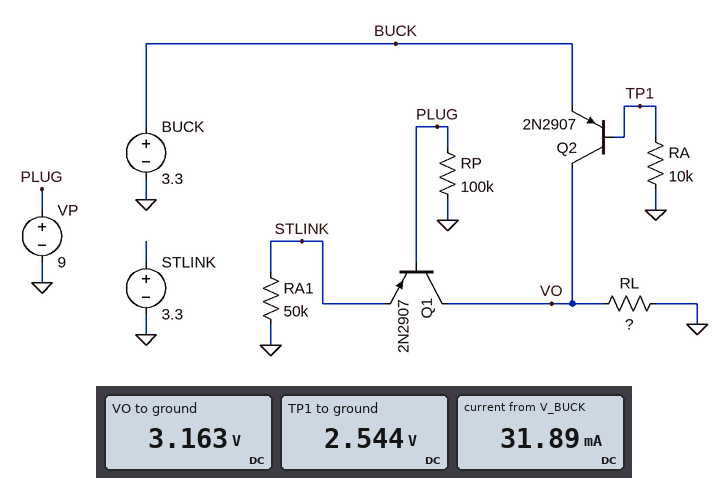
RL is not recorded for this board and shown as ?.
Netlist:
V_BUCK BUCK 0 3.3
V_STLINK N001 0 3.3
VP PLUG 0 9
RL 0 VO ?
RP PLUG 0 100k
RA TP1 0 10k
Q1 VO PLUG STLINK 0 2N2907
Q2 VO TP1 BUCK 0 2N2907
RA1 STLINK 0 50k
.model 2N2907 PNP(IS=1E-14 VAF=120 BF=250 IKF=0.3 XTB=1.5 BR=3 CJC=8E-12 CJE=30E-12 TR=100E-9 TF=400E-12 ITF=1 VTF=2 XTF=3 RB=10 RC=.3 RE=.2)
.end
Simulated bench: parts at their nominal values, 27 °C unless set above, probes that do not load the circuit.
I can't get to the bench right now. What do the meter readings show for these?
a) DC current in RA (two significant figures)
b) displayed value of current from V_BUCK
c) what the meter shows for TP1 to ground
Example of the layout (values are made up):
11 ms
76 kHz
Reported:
250 µA
31.89 mA
2.544 V
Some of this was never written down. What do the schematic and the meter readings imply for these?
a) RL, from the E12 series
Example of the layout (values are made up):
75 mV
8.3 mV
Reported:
100 Ω
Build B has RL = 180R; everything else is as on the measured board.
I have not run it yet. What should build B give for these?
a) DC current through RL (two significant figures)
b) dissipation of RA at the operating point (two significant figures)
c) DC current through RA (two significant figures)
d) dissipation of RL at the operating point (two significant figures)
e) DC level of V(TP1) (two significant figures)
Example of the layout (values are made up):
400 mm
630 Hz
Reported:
18 mA
660 µW
260 µA
57 mW
2.6 V
